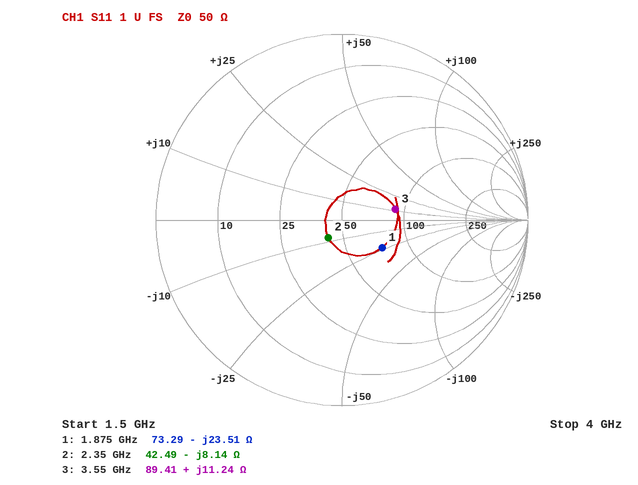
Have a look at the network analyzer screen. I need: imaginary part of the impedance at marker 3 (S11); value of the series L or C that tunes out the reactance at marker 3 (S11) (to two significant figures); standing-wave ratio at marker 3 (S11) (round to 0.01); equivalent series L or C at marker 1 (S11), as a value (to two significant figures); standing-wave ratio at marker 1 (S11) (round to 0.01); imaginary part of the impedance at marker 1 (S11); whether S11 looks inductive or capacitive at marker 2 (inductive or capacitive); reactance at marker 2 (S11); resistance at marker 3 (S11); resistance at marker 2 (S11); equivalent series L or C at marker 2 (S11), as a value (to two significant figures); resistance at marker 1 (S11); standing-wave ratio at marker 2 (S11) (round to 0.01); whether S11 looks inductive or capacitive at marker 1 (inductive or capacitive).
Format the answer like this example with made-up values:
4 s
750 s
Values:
+11.24 Ω
4.0 pF
1.83
3.6 pF
1.72
-23.51 Ω
capacitive
-8.14 Ω
89.41 Ω
42.49 Ω
8.3 pF
73.29 Ω
1.27
capacitive
